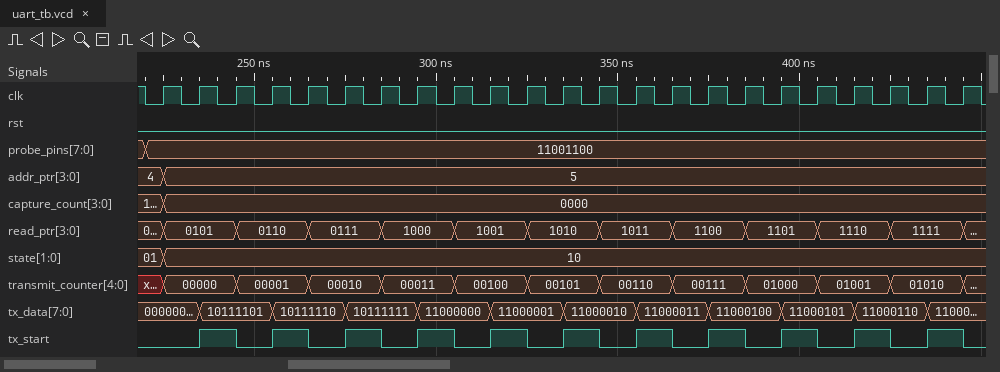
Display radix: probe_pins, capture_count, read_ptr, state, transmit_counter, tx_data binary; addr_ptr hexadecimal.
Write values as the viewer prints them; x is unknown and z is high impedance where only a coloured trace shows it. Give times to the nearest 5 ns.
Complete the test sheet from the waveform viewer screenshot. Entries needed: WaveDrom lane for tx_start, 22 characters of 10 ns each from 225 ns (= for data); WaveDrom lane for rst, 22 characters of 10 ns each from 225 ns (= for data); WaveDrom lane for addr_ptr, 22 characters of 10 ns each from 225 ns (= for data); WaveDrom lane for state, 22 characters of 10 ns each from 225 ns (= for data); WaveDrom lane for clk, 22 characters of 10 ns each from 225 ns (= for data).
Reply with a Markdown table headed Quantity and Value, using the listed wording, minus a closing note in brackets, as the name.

| Quantity | Value |
|---|---|
| WaveDrom lane for tx_start, 22 characters of 10 ns each from 225 ns | {name: 'tx_start', wave: '0101010101010101010101'} |
| WaveDrom lane for rst, 22 characters of 10 ns each from 225 ns | {name: 'rst', wave: '0.....................'} |
| WaveDrom lane for addr_ptr, 22 characters of 10 ns each from 225 ns | {name: 'addr_ptr', wave: '=.....................', data: '5'} |
| WaveDrom lane for state, 22 characters of 10 ns each from 225 ns | {name: 'state', wave: '=.....................', data: '10'} |
| WaveDrom lane for clk, 22 characters of 10 ns each from 225 ns | {name: 'clk', wave: 'p.....................'} |
